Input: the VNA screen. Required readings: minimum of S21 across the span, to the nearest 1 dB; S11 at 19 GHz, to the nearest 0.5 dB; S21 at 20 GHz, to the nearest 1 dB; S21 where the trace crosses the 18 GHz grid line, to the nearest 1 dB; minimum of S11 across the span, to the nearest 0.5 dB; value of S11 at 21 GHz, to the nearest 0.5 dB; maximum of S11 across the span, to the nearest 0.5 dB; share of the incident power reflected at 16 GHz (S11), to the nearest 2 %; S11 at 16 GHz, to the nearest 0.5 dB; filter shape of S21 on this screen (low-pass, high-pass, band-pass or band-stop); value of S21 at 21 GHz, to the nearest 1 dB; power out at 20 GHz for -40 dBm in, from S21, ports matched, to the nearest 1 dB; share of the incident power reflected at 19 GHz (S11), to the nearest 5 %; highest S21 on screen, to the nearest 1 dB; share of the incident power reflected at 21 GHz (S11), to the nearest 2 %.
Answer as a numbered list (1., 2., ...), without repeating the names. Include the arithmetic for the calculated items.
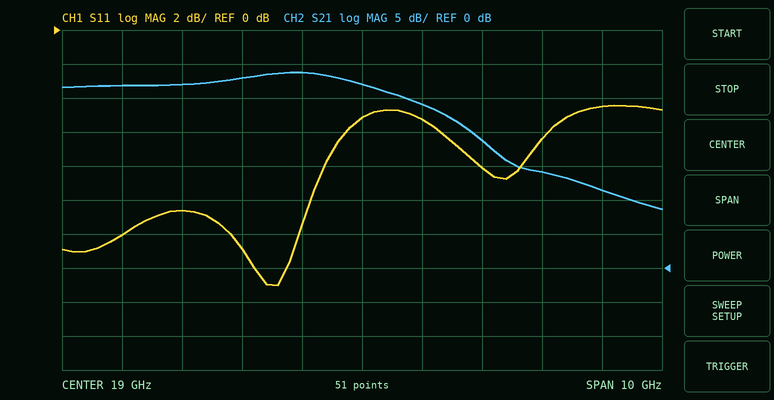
1. 9 dB
2. -5.0 dB
3. 24 dB
4. 29 dB
5. -15.0 dB
6. -8.0 dB
7. -4.5 dB
8. 10^(-10.5/10) ≈ 8.91 %, so 8 % to the nearest 2 %
9. -10.5 dB
10. low-pass
11. 19 dB
12. -40 dBm + (24 dB) = -16 dBm
13. 10^(-5/10) ≈ 31.6 %, so 30 % to the nearest 5 %
14. 29 dB
15. 10^(-8/10) ≈ 16 %
